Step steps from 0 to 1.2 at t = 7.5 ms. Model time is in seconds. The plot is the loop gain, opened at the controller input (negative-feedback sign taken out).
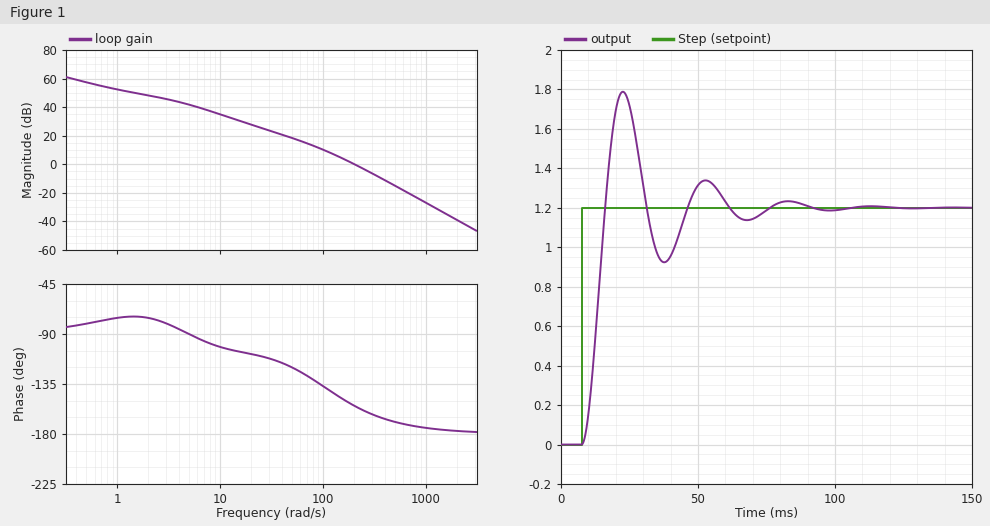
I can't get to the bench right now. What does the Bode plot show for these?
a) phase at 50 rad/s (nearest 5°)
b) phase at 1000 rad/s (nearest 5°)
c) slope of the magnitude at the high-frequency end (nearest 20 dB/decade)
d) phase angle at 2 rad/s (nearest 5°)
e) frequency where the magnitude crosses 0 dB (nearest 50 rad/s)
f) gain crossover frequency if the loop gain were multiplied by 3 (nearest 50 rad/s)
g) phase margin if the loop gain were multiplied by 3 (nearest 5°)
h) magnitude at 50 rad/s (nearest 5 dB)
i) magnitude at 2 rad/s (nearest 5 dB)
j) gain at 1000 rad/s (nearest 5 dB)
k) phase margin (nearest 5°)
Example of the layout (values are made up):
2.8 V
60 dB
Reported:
-120°
-175°
-40 dB/decade
-75°
200 rad/s
350 rad/s
15°
20 dB
50 dB
-25 dB
25°
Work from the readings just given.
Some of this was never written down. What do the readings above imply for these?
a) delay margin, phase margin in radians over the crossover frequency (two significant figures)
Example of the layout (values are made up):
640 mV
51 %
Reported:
0.0022 s
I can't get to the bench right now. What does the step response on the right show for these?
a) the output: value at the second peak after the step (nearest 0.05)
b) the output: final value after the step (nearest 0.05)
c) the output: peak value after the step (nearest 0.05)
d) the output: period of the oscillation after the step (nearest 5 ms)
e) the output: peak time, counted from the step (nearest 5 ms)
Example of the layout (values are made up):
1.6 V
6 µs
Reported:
1.35
1.20
1.80
30 ms
15 ms
